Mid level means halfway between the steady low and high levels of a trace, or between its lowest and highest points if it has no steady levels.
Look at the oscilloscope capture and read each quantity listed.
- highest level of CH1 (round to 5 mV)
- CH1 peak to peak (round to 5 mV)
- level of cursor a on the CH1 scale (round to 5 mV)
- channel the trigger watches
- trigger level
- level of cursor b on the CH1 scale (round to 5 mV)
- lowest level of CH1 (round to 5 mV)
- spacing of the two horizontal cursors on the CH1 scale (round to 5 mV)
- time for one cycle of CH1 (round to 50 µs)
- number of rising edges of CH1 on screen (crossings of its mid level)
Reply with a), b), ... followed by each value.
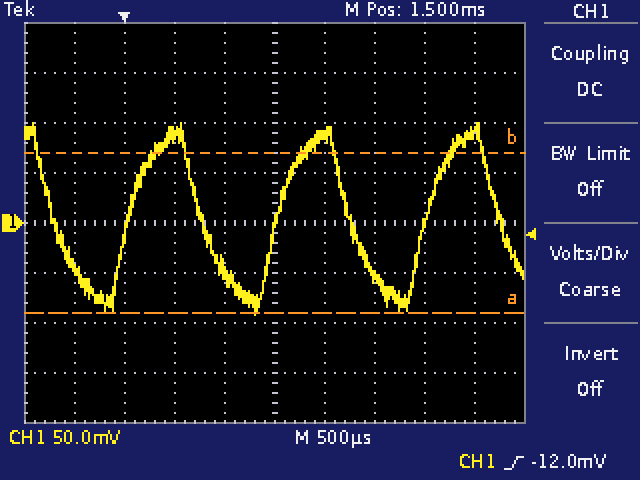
a) 100 mV
b) 190 mV
c) -90 mV
d) CH1
e) -12.0 mV
f) 70 mV
g) -90 mV
h) 160 mV
i) 1.50 ms
j) 3
